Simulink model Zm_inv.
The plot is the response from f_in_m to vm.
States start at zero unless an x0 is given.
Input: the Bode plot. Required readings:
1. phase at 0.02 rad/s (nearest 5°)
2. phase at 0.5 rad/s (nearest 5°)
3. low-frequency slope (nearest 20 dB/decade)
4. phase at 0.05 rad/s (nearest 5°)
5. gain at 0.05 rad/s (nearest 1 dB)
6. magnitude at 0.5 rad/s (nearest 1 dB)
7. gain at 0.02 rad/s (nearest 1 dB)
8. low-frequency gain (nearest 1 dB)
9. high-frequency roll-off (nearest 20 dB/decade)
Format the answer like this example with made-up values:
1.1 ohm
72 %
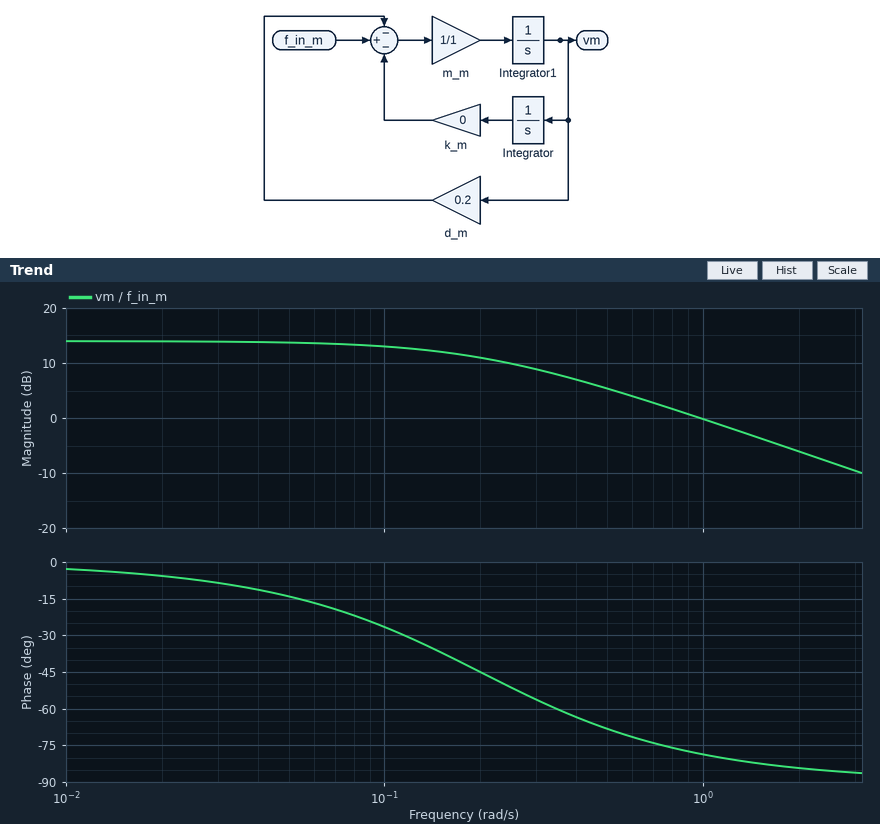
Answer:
-5°
-70°
0 dB/decade
-15°
14 dB
5 dB
14 dB
14 dB
-20 dB/decade
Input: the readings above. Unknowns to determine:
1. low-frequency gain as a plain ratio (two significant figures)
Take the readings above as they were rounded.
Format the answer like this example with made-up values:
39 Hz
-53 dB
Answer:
5.0
